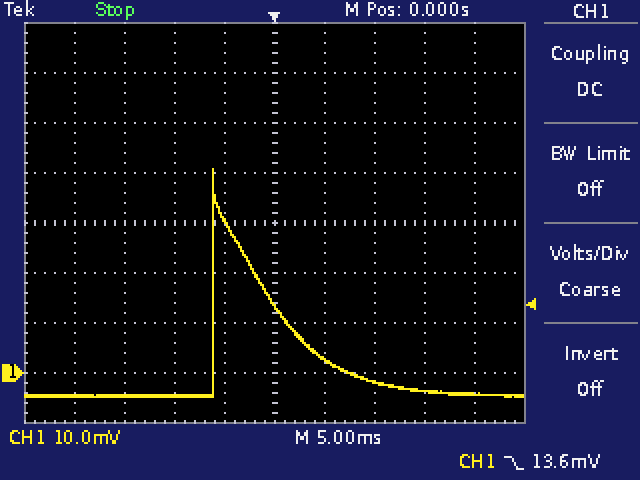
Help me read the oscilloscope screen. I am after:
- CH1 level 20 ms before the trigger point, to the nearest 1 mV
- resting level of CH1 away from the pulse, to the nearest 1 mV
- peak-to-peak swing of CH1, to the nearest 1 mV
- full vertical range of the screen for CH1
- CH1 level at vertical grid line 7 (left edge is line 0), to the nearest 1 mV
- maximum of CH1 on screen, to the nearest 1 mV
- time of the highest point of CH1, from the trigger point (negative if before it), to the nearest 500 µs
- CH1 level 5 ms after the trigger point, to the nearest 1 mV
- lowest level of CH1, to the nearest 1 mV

-5 mV
-5 mV
46 mV
80 mV
-2 mV
41 mV
-6.0 ms
3 mV
-5 mV
